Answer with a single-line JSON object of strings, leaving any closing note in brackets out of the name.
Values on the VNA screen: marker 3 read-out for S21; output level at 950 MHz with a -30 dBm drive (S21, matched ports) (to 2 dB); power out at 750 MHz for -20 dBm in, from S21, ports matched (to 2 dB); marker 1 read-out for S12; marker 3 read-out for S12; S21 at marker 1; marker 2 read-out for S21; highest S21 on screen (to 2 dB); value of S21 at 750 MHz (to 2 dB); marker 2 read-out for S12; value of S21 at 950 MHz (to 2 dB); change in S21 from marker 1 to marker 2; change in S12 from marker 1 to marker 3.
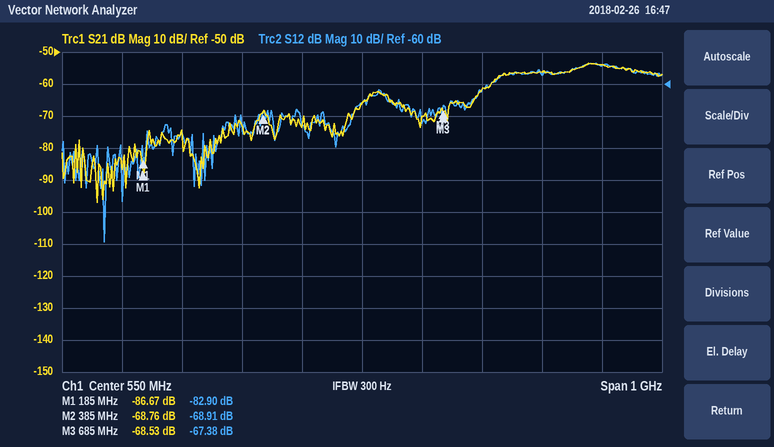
{"marker 3 read-out for S21": "-68.53 dB", "output level at 950 MHz with a -30 dBm drive (S21, matched ports)": "-84 dBm", "power out at 750 MHz for -20 dBm in, from S21, ports matched": "-82 dBm", "marker 1 read-out for S12": "-82.90 dB", "marker 3 read-out for S12": "-67.38 dB", "S21 at marker 1": "-86.67 dB", "marker 2 read-out for S21": "-68.76 dB", "highest S21 on screen": "-54 dB", "value of S21 at 750 MHz": "-62 dB", "marker 2 read-out for S12": "-68.91 dB", "value of S21 at 950 MHz": "-54 dB", "change in S21 from marker 1 to marker 2": "17.91 dB", "change in S12 from marker 1 to marker 3": "15.52 dB"}
